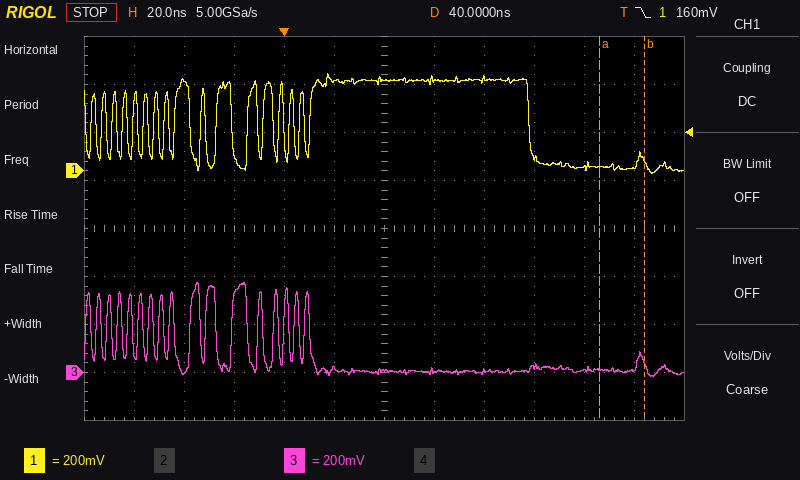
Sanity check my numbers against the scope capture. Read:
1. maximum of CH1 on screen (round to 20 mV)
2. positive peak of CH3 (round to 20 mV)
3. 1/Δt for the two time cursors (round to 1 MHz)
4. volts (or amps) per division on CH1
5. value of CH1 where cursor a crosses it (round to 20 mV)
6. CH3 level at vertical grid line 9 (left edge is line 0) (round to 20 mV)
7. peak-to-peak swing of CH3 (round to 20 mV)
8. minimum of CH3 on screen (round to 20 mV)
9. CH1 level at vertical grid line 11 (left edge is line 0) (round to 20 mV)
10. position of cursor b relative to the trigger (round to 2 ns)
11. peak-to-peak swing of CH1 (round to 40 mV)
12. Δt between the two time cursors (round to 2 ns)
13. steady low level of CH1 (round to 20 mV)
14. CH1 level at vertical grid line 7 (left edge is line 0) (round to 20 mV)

400 mV
380 mV
56 MHz
200 mV
20 mV
20 mV
400 mV
-20 mV
20 mV
+144 ns
400 mV
18 ns
20 mV
380 mV
